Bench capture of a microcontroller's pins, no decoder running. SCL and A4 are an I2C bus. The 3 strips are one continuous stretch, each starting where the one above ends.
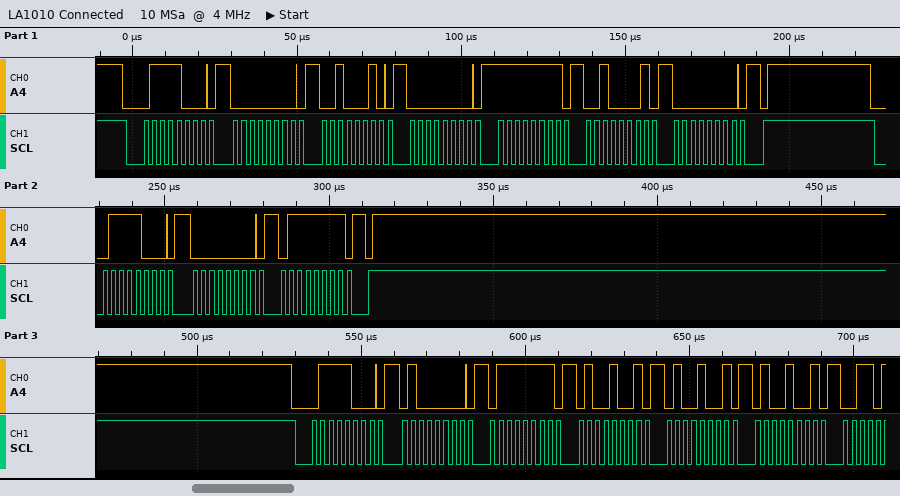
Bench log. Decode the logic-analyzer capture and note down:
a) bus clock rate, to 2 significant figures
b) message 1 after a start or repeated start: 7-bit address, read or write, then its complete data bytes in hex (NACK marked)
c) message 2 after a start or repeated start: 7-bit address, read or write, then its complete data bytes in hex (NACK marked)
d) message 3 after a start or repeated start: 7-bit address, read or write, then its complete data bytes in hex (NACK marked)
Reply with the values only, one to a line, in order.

400 kHz
0x3C write: 00 22 00 FF 21 00
0x3C write: 00 7F
0x3C write: 40 7F 49 49 49
